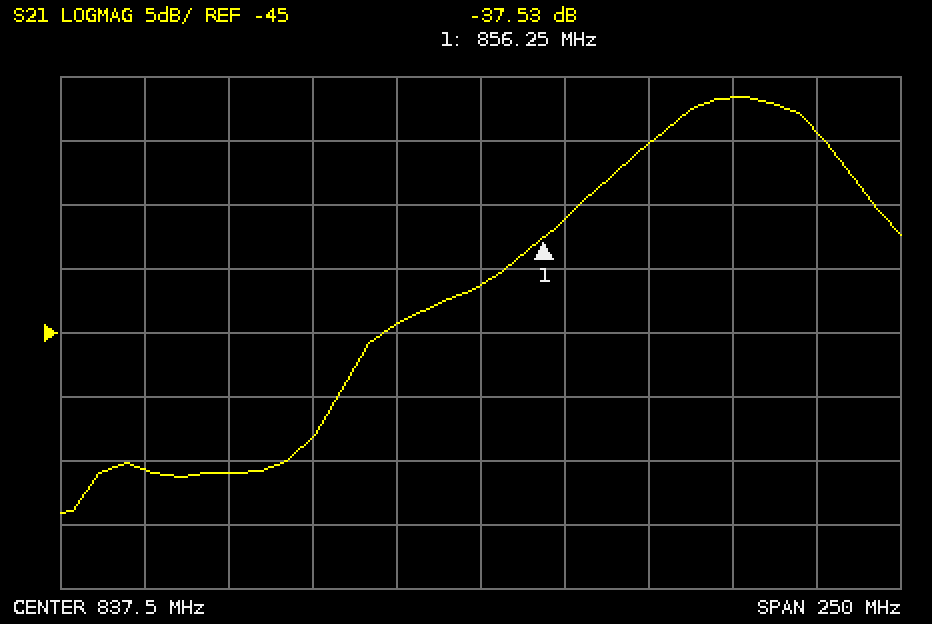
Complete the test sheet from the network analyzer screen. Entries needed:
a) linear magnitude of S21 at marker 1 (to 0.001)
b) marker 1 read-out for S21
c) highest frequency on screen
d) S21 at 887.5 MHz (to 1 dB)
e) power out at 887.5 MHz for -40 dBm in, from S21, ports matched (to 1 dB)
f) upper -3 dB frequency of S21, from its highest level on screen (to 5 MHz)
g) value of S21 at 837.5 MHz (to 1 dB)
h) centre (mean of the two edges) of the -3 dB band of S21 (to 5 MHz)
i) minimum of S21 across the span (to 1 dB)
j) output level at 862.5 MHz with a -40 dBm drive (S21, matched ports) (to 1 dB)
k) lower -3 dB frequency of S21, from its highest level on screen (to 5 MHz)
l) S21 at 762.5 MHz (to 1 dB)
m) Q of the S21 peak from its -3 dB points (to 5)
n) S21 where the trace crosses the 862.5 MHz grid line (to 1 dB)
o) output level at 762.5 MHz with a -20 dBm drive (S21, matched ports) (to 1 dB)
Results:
0.013
-37.53 dB
962.5 MHz
-30 dB
-70 dBm
940 MHz
-41 dB
915 MHz
-59 dB
-76 dBm
890 MHz
-56 dB
20
-36 dB
-76 dBm
